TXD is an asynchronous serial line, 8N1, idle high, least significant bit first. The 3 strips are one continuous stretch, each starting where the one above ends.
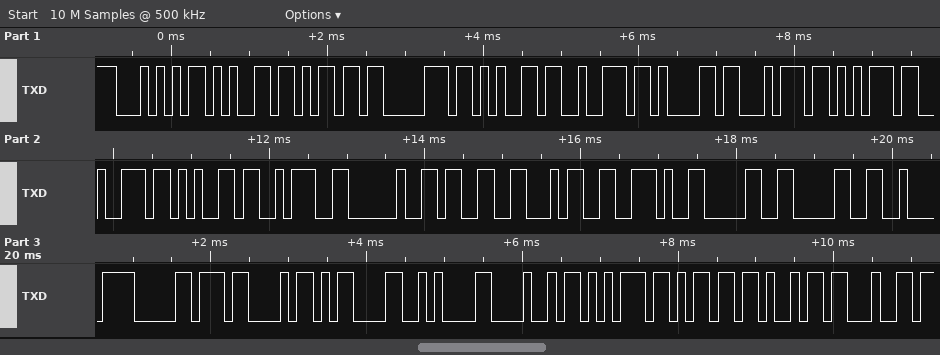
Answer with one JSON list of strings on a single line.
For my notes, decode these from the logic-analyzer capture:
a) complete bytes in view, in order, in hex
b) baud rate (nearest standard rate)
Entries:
["54 65 6D 70 65 72 61 74 75 72 65 3A 20 33 34 2E 30 30 C2 B0 43 0D 0A 48 75 6D 69 64", "9600 baud"]
